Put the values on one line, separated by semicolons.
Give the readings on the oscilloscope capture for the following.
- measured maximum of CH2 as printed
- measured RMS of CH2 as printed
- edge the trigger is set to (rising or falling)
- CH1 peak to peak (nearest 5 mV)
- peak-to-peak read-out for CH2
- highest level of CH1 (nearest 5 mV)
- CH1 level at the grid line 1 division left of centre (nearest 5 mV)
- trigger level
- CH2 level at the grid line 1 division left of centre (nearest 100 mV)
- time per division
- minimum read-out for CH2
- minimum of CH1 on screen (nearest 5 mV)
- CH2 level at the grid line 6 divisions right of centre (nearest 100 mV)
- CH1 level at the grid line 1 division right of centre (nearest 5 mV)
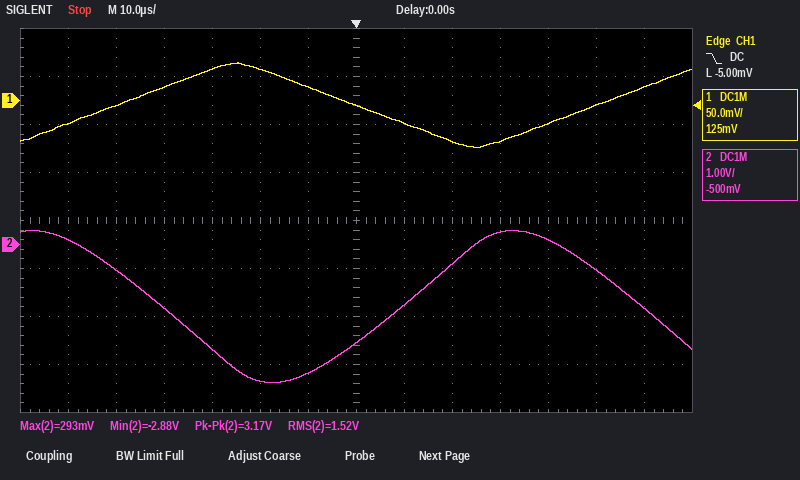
293 mV; 1.52 V; falling; 90 mV; 3.17 V; 40 mV; 15 mV; -5.00 mV; -2.7 V; 10 µs; -2.88 V; -50 mV; -1.3 V; -25 mV
